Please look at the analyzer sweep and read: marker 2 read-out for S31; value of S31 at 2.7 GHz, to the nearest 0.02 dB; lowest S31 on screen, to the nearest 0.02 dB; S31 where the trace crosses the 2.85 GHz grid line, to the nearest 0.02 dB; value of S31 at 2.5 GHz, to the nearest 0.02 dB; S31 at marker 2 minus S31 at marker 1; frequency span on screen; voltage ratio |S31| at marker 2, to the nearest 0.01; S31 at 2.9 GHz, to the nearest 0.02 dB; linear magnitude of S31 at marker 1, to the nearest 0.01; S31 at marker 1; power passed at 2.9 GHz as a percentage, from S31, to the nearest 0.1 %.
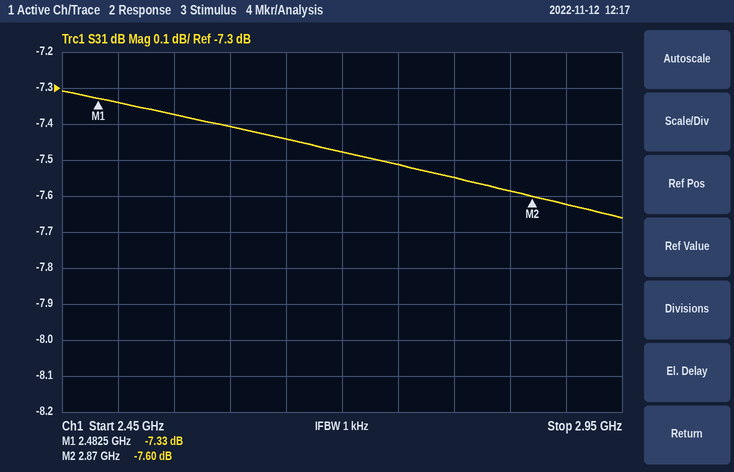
-7.60 dB
-7.48 dB
-7.66 dB
-7.58 dB
-7.34 dB
-0.27 dB
500 MHz
0.42
-7.62 dB
0.43
-7.33 dB
17.3 %
